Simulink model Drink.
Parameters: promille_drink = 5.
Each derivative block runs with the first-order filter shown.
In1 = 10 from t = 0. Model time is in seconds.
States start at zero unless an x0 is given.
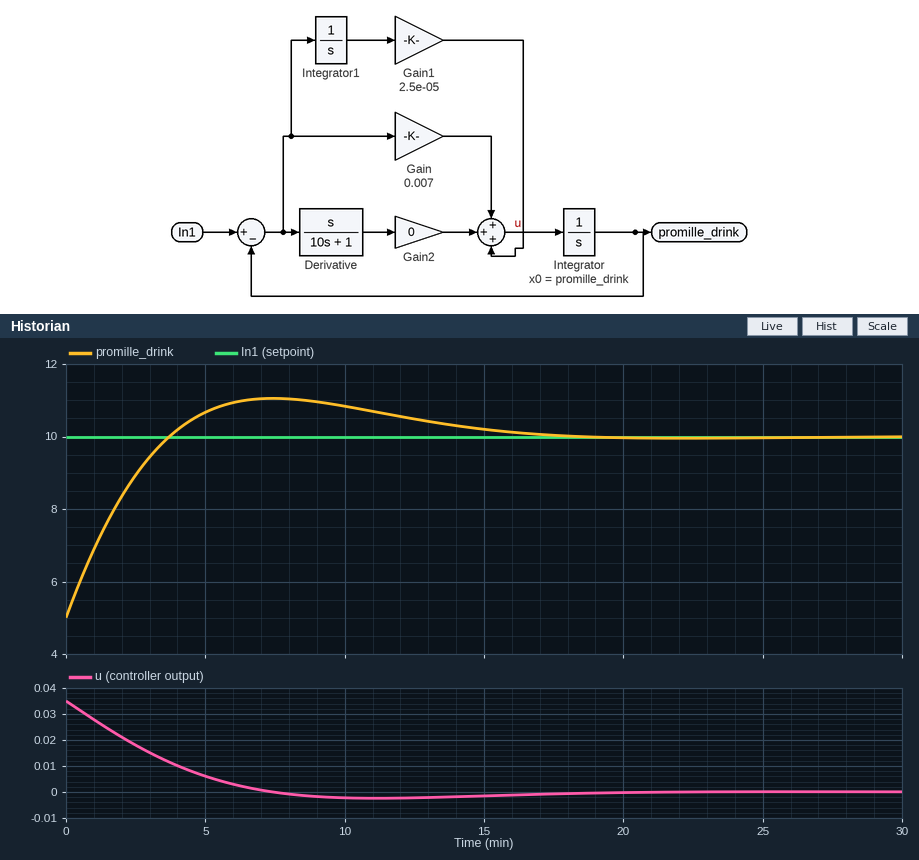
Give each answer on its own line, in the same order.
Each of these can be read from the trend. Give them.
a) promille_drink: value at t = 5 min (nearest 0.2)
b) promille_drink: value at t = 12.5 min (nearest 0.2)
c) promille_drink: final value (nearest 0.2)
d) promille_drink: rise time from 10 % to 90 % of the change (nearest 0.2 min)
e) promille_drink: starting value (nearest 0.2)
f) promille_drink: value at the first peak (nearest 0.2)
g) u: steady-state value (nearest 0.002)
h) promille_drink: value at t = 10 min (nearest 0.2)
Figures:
10.6
10.4
10.0
2.8 min
5.0
11.0
0.000
10.8
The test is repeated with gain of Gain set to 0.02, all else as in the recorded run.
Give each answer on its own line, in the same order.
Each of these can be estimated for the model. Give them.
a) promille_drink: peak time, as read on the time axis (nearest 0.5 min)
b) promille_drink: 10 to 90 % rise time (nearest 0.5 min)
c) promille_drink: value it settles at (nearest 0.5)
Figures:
5.0 min
1.5 min
10.0
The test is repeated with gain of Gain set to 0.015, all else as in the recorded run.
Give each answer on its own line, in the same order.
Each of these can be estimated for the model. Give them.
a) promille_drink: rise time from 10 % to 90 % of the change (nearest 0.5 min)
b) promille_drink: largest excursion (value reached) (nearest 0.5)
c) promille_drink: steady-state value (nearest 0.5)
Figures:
2.0 min
10.5
10.0
